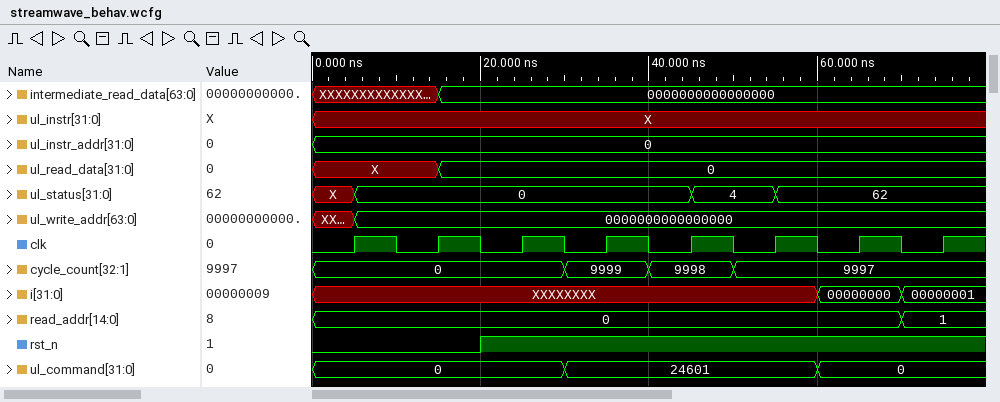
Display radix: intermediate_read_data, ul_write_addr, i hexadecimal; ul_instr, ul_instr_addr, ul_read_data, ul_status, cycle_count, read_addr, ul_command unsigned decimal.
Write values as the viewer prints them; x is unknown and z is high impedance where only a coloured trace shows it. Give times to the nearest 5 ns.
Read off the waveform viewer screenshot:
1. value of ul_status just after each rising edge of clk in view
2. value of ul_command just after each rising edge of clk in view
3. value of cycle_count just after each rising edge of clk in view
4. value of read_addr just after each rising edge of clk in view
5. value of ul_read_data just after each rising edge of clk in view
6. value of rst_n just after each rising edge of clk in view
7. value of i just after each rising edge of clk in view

0, 0, 0, 0, 4, 62, 62, 62
0, 0, 0, 24601, 24601, 24601, 0, 0
0, 0, 0, 9999, 9998, 9997, 9997, 9997
0, 0, 0, 0, 0, 0, 0, 1
X, 0, 0, 0, 0, 0, 0, 0
0 0 1 1 1 1 1 1
XXXXXXXX, XXXXXXXX, XXXXXXXX, XXXXXXXX, XXXXXXXX, XXXXXXXX, 00000000, 00000001
